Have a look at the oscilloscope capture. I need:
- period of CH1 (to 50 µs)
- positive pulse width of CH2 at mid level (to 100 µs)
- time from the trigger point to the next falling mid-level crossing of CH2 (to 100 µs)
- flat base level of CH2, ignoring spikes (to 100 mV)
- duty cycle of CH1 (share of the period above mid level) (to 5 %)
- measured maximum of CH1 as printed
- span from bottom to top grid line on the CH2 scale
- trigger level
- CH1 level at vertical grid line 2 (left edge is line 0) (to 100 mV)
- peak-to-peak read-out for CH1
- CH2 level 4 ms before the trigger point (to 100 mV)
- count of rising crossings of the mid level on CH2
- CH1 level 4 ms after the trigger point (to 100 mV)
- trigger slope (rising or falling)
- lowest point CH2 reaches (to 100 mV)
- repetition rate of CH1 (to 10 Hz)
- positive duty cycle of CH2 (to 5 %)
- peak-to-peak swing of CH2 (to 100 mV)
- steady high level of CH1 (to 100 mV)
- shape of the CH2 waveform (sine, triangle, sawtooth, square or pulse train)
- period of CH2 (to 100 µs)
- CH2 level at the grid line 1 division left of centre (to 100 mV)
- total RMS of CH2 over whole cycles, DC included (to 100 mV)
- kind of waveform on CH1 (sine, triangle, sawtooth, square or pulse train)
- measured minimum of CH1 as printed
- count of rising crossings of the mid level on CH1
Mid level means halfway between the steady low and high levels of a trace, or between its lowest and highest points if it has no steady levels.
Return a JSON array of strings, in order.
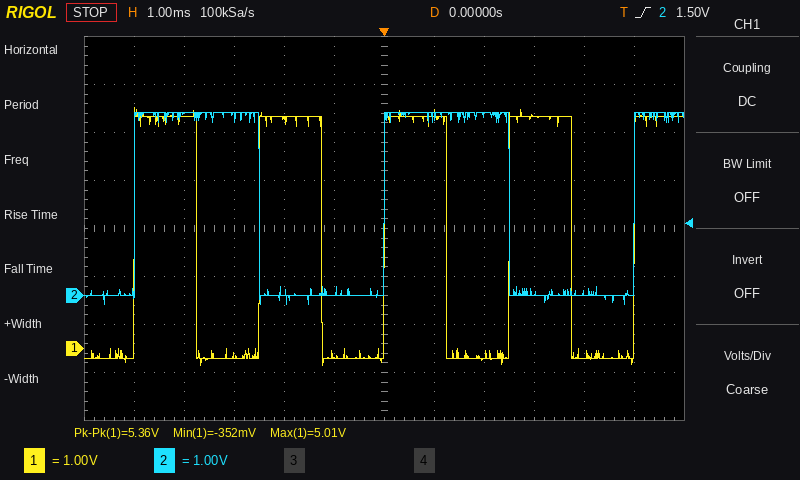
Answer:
["2.50 ms", "2.5 ms", "2.5 ms", "0.0 V", "50 %", "5.01 V", "8 V", "1.50 V", "4.8 V", "5.36 V", "3.8 V", "3", "-100 mV", "rising", "-200 mV", "400 Hz", "50 %", "4.0 V", "4.8 V", "square", "5.0 ms", "100 mV", "2.7 V", "square", "-352 mV", "5"]
